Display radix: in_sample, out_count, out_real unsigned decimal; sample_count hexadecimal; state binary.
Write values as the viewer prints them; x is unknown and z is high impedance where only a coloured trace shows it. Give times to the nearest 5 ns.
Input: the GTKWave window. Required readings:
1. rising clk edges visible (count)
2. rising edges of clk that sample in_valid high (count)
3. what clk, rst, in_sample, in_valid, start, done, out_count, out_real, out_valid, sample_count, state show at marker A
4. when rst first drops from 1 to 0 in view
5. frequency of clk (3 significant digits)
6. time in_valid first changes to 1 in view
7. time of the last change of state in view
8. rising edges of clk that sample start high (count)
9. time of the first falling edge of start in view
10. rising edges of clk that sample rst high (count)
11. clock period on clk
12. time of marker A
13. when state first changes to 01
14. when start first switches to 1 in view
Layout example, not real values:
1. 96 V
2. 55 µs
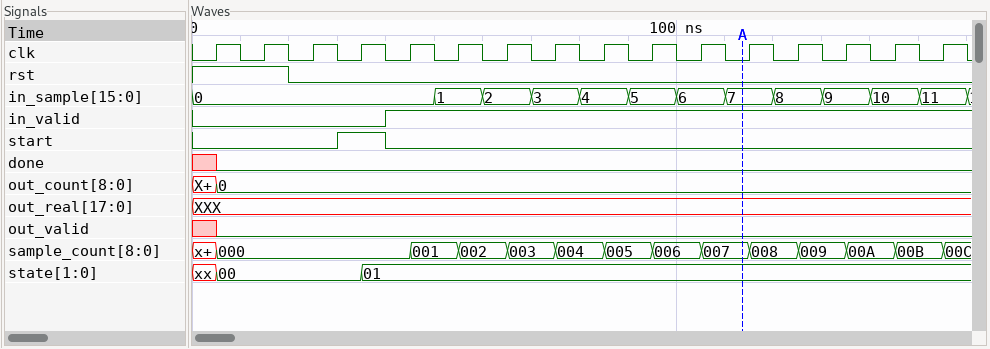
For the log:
1. 16
2. 12
3. clk=0, rst=0, in_sample=7, in_valid=1, start=0, done=0, out_count=0, out_real=XXX, out_valid=0, sample_count=007, state=01
4. 20 ns
5. 100 MHz
6. 40 ns
7. 35 ns
8. 1
9. 40 ns
10. 2
11. 10 ns
12. 115 ns
13. 35 ns
14. 30 ns
